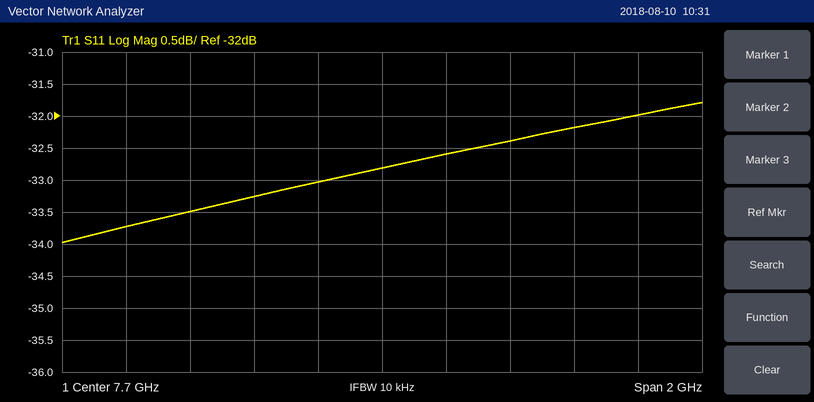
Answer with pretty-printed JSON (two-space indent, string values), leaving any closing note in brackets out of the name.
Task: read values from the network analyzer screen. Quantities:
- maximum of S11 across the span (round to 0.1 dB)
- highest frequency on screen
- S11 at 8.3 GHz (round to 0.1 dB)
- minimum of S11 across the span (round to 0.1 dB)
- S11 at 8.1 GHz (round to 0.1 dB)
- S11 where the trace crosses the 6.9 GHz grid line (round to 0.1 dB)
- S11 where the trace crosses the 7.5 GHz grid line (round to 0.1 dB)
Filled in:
{
  "maximum of S11 across the span": "-31.8 dB",
  "highest frequency on screen": "8.7 GHz",
  "S11 at 8.3 GHz": "-32.2 dB",
  "minimum of S11 across the span": "-34.0 dB",
  "S11 at 8.1 GHz": "-32.4 dB",
  "S11 where the trace crosses the 6.9 GHz grid line": "-33.7 dB",
  "S11 where the trace crosses the 7.5 GHz grid line": "-33.0 dB"
}
